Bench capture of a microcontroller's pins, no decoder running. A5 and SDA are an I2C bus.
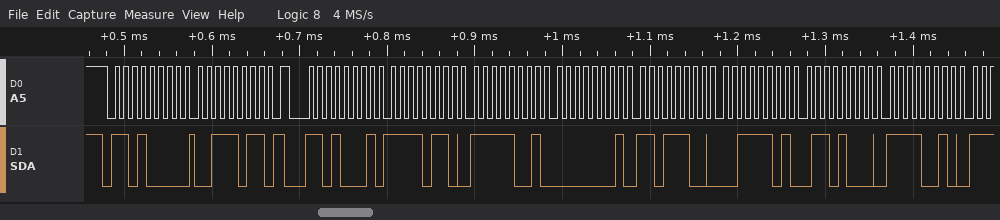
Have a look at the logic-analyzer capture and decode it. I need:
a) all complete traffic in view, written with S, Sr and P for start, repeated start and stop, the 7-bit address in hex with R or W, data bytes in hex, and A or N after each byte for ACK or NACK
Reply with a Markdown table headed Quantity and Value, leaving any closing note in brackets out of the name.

| Quantity | Value |
|---|---|
| all complete traffic in view, written with S, Sr and P for start, repeated start and stop, the 7-bit address in hex with R or W, data bytes in hex, and A or N after each byte for ACK or NACK | S 68W A 3B A Sr 68R A F6 A F9 A 01 A DC A 3D A 68 A F2 A |
